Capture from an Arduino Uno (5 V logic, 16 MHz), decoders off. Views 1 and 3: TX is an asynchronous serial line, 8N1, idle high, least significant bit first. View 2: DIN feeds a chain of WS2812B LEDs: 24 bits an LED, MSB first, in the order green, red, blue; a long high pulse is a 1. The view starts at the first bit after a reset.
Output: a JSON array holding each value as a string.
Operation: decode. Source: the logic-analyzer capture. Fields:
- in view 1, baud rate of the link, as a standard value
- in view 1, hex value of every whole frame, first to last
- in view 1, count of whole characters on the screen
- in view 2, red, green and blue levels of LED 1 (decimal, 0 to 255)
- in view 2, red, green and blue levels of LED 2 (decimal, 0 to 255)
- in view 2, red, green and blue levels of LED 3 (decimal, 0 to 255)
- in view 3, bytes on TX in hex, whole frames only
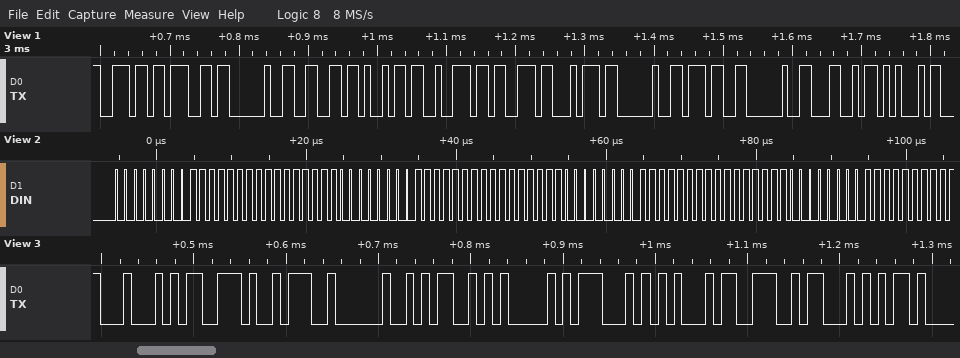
["115200 baud", "6E 67 20 66 69 72 73 74 20 37 20 4C 45", "13", "255, 0, 255", "255, 0, 255", "255, 0, 255", "44 73 3A 20 4D 41 47 45 4E 54"]
